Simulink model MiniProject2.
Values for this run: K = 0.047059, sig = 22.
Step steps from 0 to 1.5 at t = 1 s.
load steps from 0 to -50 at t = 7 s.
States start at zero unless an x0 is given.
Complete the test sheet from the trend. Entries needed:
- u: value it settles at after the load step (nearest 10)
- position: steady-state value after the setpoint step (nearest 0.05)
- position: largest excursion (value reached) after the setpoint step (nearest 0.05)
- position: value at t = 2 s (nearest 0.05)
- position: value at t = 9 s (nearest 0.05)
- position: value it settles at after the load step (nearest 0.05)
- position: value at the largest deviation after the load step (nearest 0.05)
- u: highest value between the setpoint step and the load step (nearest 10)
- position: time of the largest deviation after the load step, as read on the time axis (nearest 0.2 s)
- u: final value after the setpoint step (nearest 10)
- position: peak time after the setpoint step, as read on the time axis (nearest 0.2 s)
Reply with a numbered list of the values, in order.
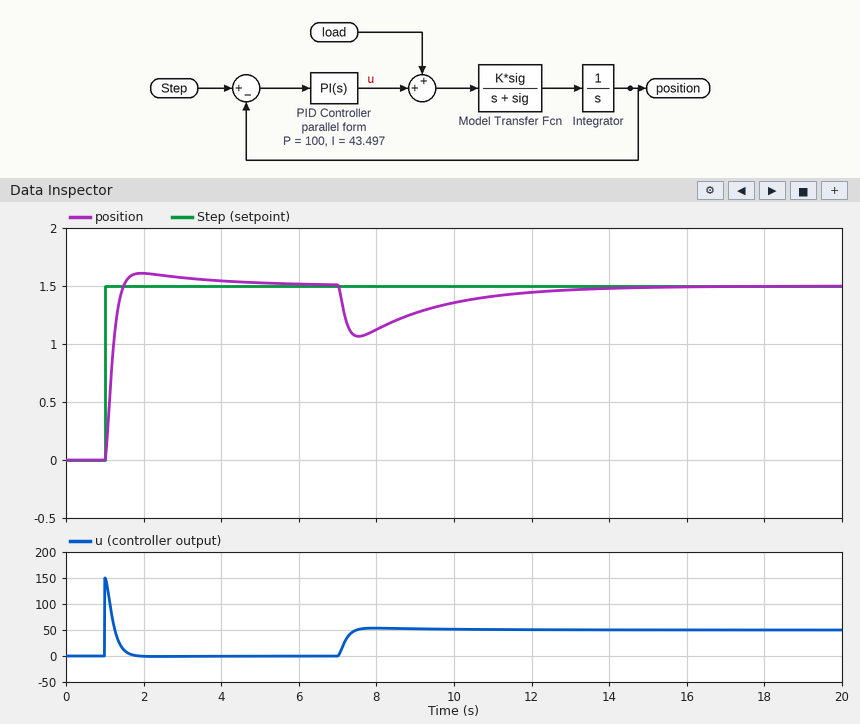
1. 50
2. 1.50
3. 1.60
4. 1.60
5. 1.25
6. 1.50
7. 1.05
8. 150
9. 7.6 s
10. 0
11. 2.0 s
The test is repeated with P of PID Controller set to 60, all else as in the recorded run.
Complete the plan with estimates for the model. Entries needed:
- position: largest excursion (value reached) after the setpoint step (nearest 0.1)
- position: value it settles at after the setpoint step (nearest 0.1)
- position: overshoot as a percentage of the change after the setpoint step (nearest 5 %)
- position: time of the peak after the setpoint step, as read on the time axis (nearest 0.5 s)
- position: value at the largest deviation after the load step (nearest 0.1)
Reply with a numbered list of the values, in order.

1. 1.7
2. 1.5
3. 15 %
4. 2.5 s
5. 0.9
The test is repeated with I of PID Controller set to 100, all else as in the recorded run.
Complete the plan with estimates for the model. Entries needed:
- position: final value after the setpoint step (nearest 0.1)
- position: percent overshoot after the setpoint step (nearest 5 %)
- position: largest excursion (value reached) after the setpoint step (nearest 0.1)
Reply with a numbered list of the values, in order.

1. 1.5
2. 15 %
3. 1.7
